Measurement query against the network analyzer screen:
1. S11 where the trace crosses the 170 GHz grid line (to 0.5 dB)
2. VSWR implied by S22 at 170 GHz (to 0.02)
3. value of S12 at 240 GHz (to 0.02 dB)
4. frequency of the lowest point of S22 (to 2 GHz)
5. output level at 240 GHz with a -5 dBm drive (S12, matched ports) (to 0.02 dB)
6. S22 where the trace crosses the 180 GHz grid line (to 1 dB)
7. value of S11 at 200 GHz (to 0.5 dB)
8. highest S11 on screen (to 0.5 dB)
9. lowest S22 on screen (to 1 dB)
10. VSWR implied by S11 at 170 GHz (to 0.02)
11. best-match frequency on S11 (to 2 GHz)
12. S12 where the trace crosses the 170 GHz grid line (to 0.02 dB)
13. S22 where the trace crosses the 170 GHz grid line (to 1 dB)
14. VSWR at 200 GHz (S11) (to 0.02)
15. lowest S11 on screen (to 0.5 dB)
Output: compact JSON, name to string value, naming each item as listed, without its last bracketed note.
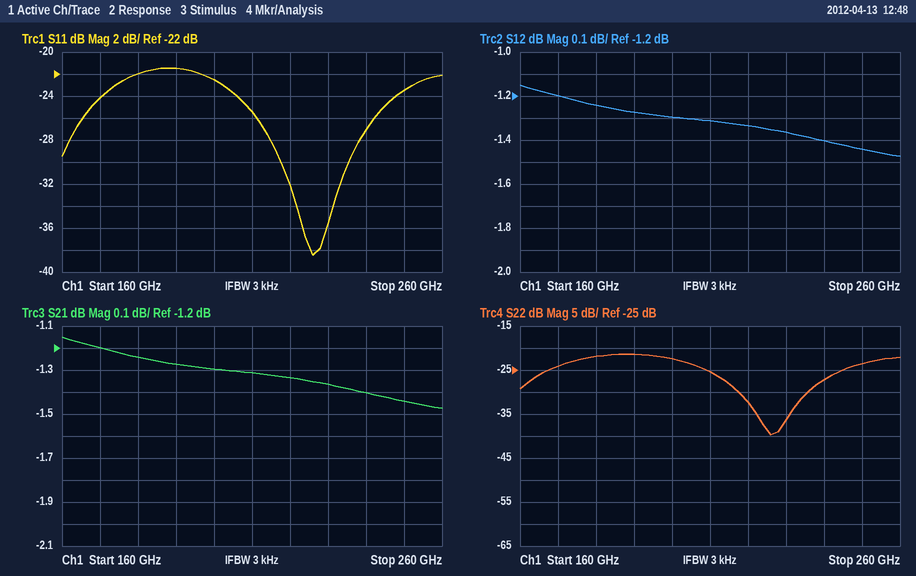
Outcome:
{"S11 where the trace crosses the 170 GHz grid line": "-24.0 dB", "VSWR implied by S22 at 170 GHz": "1.14", "value of S12 at 240 GHz": "-1.40 dB", "frequency of the lowest point of S22": "226 GHz", "output level at 240 GHz with a -5 dBm drive (S12, matched ports)": "-6.40 dBm", "S22 where the trace crosses the 180 GHz grid line": "-22 dB", "value of S11 at 200 GHz": "-22.5 dB", "highest S11 on screen": "-21.5 dB", "lowest S22 on screen": "-40 dB", "VSWR implied by S11 at 170 GHz": "1.14", "best-match frequency on S11": "226 GHz", "S12 where the trace crosses the 170 GHz grid line": "-1.20 dB", "S22 where the trace crosses the 170 GHz grid line": "-24 dB", "VSWR at 200 GHz (S11)": "1.16", "lowest S11 on screen": "-38.5 dB"}
